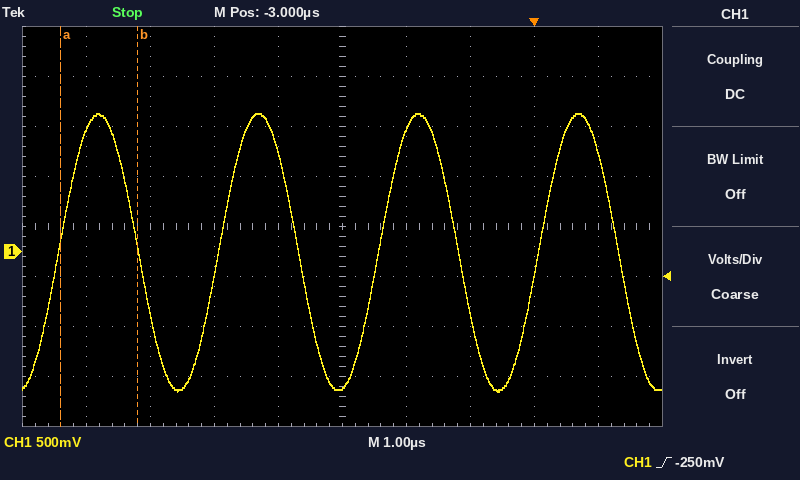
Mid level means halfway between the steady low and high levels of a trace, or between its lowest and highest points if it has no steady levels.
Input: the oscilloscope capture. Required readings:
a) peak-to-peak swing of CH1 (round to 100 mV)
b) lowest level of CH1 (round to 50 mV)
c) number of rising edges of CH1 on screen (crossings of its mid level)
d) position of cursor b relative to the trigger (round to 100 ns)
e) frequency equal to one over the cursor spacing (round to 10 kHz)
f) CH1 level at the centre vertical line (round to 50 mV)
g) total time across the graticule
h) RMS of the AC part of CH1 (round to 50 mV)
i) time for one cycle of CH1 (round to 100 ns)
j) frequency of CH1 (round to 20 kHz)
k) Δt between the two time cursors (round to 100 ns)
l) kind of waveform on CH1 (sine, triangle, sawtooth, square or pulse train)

2.80 V
-1.40 V
4
-6.2 µs
830 kHz
-1.35 V
10 µs
1.00 V
2.5 µs
400 kHz
1.2 µs
sine
